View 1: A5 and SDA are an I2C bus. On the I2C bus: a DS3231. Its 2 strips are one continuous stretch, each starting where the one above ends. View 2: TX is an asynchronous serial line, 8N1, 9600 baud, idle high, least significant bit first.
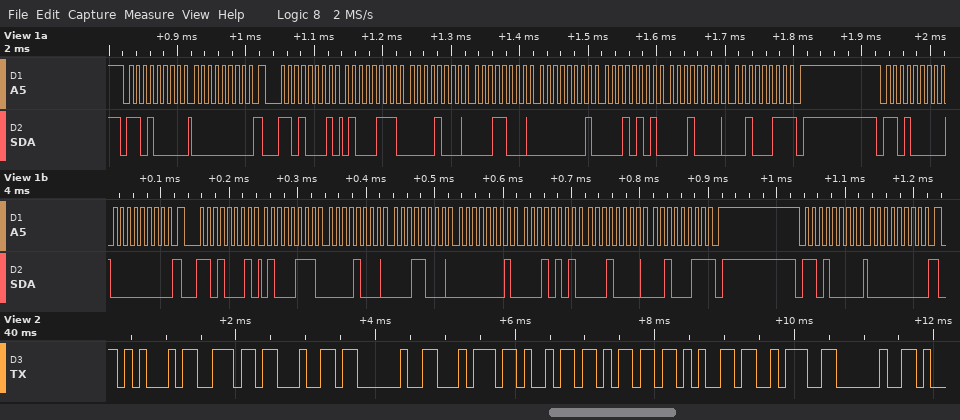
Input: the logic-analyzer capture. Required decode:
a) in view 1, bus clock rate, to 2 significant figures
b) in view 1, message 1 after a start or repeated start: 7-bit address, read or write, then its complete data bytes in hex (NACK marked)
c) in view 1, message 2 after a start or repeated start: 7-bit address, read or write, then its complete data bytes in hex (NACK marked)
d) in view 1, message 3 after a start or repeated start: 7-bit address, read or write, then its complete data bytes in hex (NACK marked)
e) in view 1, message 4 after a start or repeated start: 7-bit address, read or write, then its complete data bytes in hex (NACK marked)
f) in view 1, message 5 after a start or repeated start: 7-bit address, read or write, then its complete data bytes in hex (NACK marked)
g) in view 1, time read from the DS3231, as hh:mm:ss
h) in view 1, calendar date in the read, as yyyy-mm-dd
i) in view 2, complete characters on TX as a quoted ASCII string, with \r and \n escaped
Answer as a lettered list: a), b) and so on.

a) 100 kHz
b) 0x68 write: 00
c) 0x68 read: 47 08 18 01 15 10 23 NACK
d) 0x68 write: 00
e) 0x68 read: 47 08 18 01 15 10 23 NACK
f) 0x68 write: 00
g) 18:08:47
h) 2023-10-15
i) "End time: "
